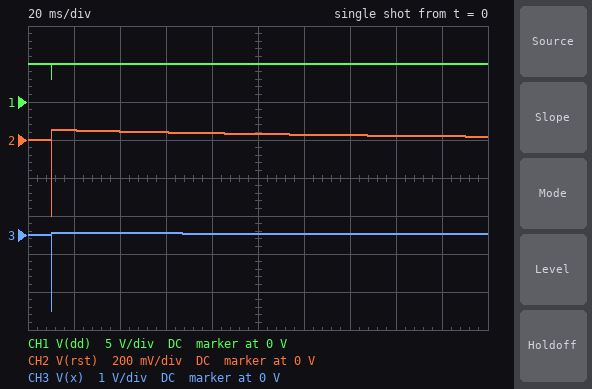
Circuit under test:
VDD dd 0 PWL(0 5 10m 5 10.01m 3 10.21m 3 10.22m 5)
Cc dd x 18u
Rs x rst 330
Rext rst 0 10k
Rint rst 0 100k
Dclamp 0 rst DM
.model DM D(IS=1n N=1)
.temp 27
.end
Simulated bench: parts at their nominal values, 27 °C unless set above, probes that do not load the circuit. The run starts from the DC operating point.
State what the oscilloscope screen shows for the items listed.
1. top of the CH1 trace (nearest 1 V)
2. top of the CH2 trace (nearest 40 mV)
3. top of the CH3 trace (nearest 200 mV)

5 V
40 mV
0 V
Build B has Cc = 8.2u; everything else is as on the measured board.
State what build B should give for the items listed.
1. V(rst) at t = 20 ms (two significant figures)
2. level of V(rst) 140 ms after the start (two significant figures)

100 mV
21 mV
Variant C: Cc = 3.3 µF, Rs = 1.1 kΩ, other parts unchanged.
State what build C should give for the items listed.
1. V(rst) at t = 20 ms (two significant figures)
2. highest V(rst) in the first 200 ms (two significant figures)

61 mV
81 mV
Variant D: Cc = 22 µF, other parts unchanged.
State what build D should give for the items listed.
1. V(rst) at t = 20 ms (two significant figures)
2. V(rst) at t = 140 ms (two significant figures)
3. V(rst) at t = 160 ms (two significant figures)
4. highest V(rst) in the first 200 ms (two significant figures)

42 mV
23 mV
21 mV
44 mV
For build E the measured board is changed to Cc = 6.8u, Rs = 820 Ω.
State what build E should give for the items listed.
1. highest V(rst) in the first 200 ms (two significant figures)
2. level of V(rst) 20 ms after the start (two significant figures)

55 mV
47 mV
